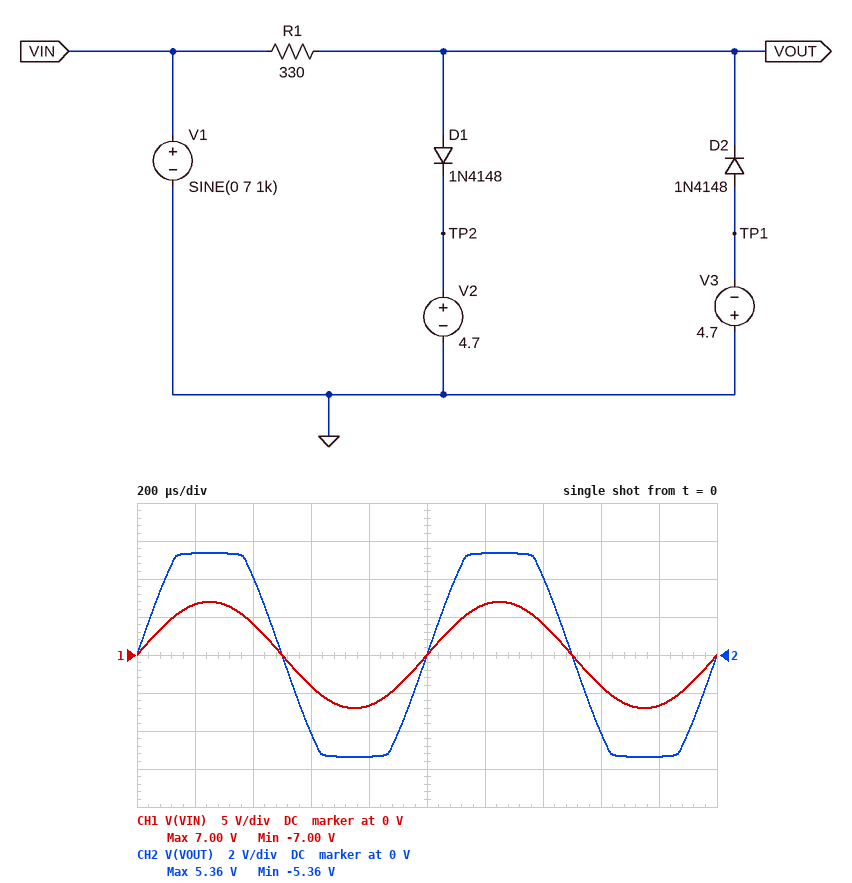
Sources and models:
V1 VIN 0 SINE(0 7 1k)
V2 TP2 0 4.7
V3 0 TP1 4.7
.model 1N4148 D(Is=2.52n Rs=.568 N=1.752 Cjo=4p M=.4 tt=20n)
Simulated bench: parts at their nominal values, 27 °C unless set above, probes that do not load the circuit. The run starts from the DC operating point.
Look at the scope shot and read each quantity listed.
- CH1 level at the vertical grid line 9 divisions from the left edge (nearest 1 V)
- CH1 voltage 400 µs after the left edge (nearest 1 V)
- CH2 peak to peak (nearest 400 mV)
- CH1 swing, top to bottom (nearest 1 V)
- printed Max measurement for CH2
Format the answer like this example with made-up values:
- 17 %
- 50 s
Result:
- -7 V
- 4 V
- 10.8 V
- 14 V
- 5.36 V
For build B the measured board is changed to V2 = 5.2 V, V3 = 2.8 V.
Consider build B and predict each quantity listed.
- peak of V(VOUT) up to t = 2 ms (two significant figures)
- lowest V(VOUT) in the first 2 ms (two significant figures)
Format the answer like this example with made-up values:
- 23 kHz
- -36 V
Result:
- 5.8 V
- -3.5 V
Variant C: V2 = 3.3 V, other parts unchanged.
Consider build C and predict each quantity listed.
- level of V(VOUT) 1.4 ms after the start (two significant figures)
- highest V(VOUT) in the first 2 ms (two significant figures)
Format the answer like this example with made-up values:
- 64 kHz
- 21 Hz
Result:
- 3.9 V
- 4.0 V
